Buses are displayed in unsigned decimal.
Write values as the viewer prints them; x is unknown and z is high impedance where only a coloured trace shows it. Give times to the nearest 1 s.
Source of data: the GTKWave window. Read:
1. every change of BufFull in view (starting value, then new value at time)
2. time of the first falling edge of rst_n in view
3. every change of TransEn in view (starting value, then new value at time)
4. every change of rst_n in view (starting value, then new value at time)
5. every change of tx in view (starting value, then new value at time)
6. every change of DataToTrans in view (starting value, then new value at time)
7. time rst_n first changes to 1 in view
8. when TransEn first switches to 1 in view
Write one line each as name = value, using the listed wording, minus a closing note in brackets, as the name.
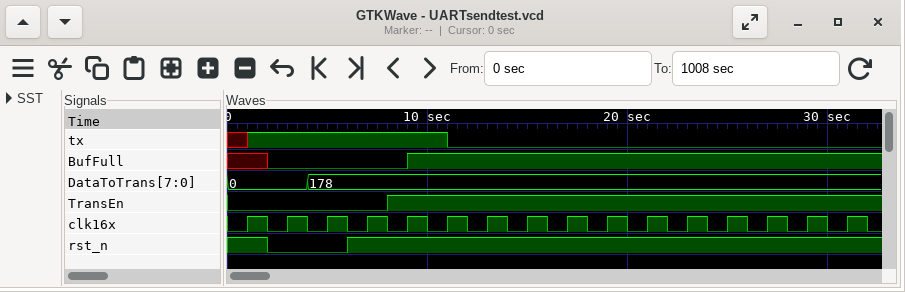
every change of BufFull in view = x, 0 at 2 s, 1 at 9 s
time of the first falling edge of rst_n in view = 2 s
every change of TransEn in view = 0, 1 at 8 s
every change of rst_n in view = 1, 0 at 2 s, 1 at 6 s
every change of tx in view = x, 1 at 1 s, 0 at 11 s
every change of DataToTrans in view = 0, 178 at 4 s
time rst_n first changes to 1 in view = 6 s
when TransEn first switches to 1 in view = 8 s
